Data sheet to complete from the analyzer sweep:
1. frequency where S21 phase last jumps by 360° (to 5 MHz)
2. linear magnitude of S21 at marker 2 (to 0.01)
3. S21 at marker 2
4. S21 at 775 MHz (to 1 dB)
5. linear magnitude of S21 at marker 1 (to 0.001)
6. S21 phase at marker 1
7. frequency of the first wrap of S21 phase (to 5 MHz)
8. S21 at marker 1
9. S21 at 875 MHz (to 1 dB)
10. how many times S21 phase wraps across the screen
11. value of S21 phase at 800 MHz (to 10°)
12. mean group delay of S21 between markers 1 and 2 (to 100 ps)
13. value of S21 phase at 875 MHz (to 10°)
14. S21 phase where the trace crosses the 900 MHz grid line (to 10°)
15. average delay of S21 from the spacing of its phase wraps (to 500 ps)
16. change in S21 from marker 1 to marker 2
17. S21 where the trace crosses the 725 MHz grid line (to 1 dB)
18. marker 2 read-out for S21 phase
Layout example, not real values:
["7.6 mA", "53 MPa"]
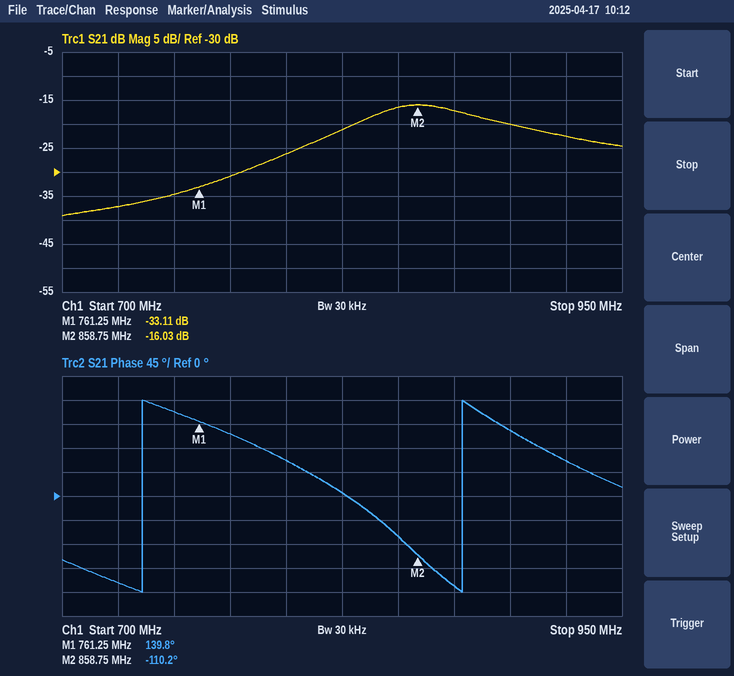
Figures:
["880 MHz", "0.16", "-16.03 dB", "-31 dB", "0.022", "139.8°", "735 MHz", "-33.11 dB", "-17 dB", "2", "70°", "7.1 ns", "-170°", "120°", "7.0 ns", "17.08 dB", "-37 dB", "-110.2°"]
